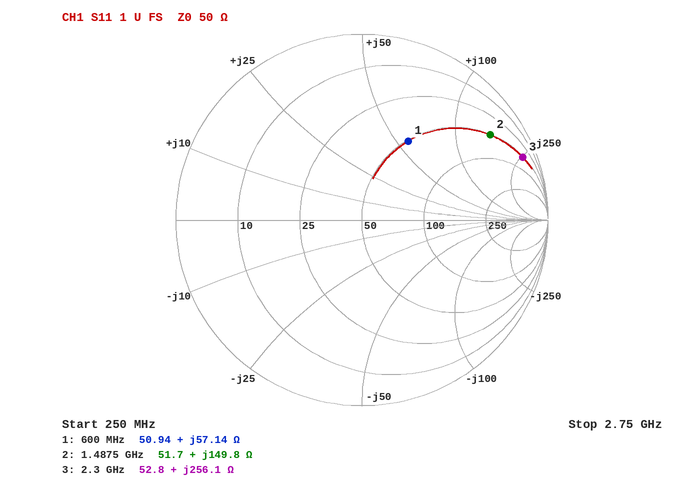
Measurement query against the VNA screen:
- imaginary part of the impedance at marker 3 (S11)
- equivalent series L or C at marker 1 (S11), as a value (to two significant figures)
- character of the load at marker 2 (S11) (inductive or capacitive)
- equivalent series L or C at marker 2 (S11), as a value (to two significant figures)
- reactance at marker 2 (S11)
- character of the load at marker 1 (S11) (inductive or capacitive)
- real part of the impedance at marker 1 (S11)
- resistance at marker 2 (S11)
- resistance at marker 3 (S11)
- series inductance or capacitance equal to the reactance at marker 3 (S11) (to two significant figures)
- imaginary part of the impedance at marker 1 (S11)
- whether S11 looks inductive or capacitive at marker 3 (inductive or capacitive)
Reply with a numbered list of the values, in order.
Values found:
1. +256.1 Ω
2. 15 nH
3. inductive
4. 16 nH
5. +149.8 Ω
6. inductive
7. 50.94 Ω
8. 51.7 Ω
9. 52.8 Ω
10. 18 nH
11. +57.14 Ω
12. inductive
